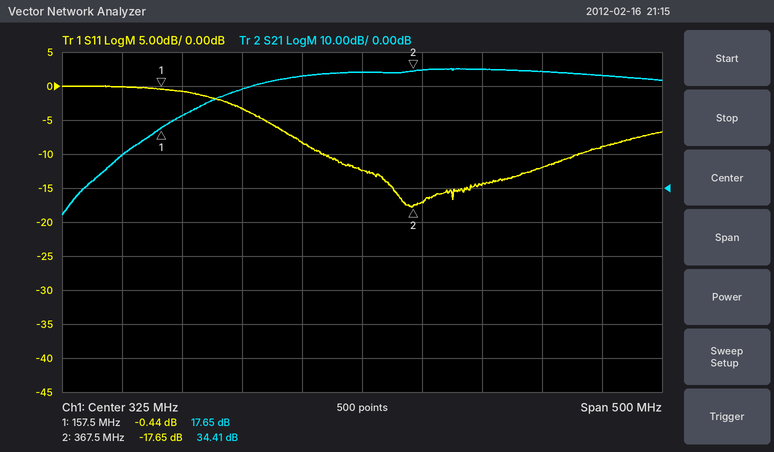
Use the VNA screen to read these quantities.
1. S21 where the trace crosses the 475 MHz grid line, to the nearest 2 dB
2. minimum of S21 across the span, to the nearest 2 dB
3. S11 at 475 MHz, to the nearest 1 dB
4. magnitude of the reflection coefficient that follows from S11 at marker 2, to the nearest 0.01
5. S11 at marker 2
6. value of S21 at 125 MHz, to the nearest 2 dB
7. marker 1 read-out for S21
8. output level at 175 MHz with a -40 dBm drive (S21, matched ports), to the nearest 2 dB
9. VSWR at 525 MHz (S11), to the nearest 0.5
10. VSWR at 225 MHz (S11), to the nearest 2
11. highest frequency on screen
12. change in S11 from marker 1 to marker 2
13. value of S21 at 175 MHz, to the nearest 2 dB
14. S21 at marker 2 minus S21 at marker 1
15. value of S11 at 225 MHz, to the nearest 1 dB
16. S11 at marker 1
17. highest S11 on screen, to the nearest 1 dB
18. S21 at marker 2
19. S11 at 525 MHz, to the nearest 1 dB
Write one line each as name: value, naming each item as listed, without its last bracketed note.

S21 where the trace crosses the 475 MHz grid line, to the nearest 2 dB: 34 dB
minimum of S21 across the span, to the nearest 2 dB: -8 dB
S11 at 475 MHz, to the nearest 1 dB: -12 dB
magnitude of the reflection coefficient that follows from S11 at marker 2, to the nearest 0.01: 0.13
S11 at marker 2: -17.65 dB
value of S21 at 125 MHz, to the nearest 2 dB: 10 dB
marker 1 read-out for S21: 17.65 dB
output level at 175 MHz with a -40 dBm drive (S21, matched ports), to the nearest 2 dB: -18 dBm
VSWR at 525 MHz (S11), to the nearest 0.5: 2.0
VSWR at 225 MHz (S11), to the nearest 2: 6
highest frequency on screen: 575 MHz
change in S11 from marker 1 to marker 2: -17.21 dB
value of S21 at 175 MHz, to the nearest 2 dB: 22 dB
S21 at marker 2 minus S21 at marker 1: 16.76 dB
value of S11 at 225 MHz, to the nearest 1 dB: -3 dB
S11 at marker 1: -0.44 dB
highest S11 on screen, to the nearest 1 dB: 0 dB
S21 at marker 2: 34.41 dB
S11 at 525 MHz, to the nearest 1 dB: -9 dB
